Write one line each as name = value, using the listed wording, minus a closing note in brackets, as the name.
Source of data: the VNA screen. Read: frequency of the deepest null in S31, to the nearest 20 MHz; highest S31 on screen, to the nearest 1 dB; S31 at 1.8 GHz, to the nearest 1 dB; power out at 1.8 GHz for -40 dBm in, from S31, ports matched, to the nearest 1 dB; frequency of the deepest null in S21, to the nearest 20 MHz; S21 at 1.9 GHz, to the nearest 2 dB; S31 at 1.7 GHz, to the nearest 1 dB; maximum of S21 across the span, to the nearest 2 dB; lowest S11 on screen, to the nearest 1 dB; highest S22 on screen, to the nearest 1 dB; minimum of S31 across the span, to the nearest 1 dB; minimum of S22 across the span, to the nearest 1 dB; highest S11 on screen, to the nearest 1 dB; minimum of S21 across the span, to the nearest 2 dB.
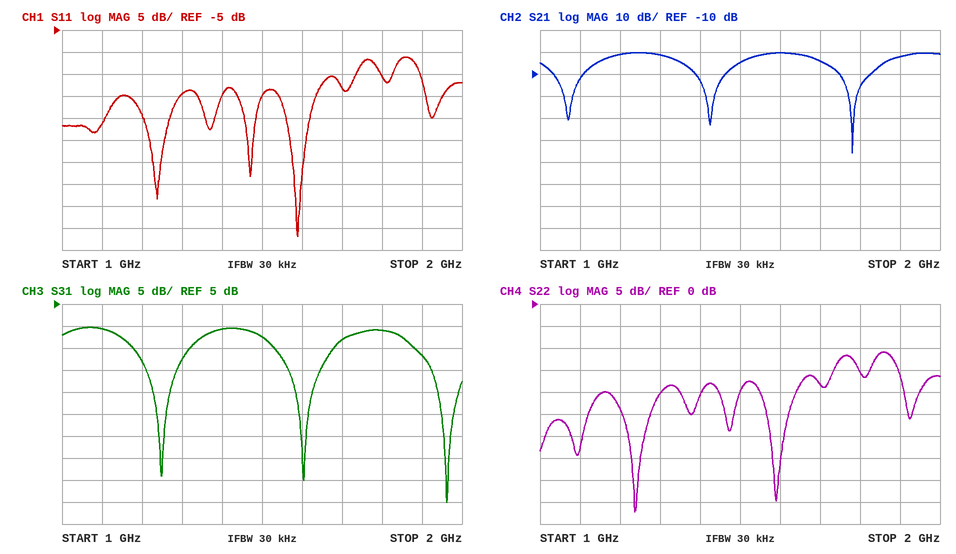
frequency of the deepest null in S31, to the nearest 20 MHz = 1.96 GHz
highest S31 on screen, to the nearest 1 dB = 0 dB
S31 at 1.8 GHz, to the nearest 1 dB = -1 dB
power out at 1.8 GHz for -40 dBm in, from S31, ports matched, to the nearest 1 dB = -41 dBm
frequency of the deepest null in S21, to the nearest 20 MHz = 1.78 GHz
S21 at 1.9 GHz, to the nearest 2 dB = -2 dB
S31 at 1.7 GHz, to the nearest 1 dB = -3 dB
maximum of S21 across the span, to the nearest 2 dB = 0 dB
lowest S11 on screen, to the nearest 1 dB = -52 dB
highest S22 on screen, to the nearest 1 dB = -11 dB
minimum of S31 across the span, to the nearest 1 dB = -40 dB
minimum of S22 across the span, to the nearest 1 dB = -47 dB
highest S11 on screen, to the nearest 1 dB = -11 dB
minimum of S21 across the span, to the nearest 2 dB = -46 dB
